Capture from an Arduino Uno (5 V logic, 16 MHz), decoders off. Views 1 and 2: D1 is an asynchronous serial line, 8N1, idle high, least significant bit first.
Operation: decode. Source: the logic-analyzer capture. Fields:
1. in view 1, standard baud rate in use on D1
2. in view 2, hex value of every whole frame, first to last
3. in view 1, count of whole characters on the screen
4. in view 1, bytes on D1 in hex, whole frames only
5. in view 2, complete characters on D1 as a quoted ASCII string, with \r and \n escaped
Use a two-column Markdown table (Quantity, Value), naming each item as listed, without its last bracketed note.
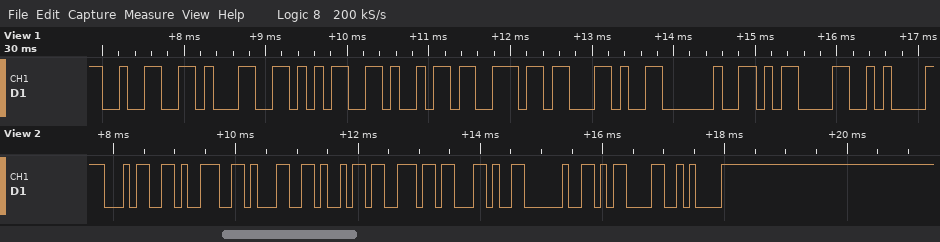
| Quantity | Value |
|---|---|
| in view 1, standard baud rate in use on D1 | 9600 baud |
| in view 2, hex value of every whole frame, first to last | 34 39 31 69 6E 2C 20 0D 0A |
| in view 1, count of whole characters on the screen | 9 |
| in view 1, bytes on D1 in hex, whole frames only | 0x32 0x31 0x35 0x69 0x6E 0x2C 0x20 0x0D 0x0A |
| in view 2, complete characters on D1 as a quoted ASCII string, with \r and \n escaped | "491in, \r\n" |
